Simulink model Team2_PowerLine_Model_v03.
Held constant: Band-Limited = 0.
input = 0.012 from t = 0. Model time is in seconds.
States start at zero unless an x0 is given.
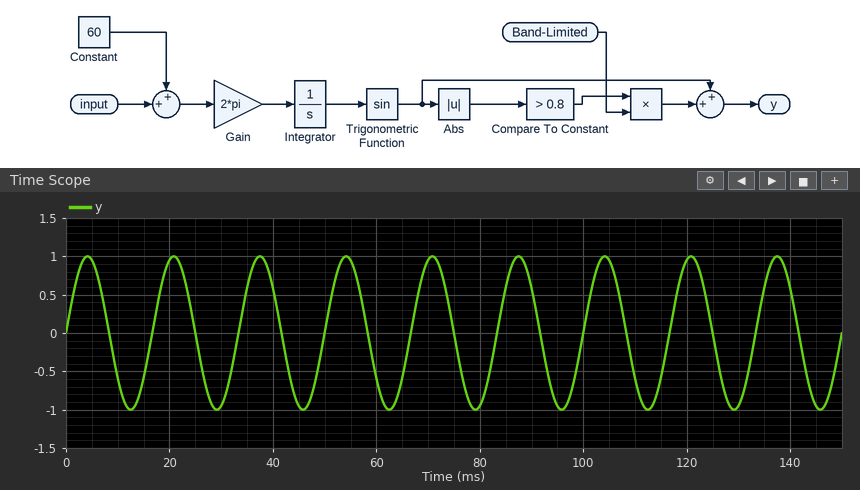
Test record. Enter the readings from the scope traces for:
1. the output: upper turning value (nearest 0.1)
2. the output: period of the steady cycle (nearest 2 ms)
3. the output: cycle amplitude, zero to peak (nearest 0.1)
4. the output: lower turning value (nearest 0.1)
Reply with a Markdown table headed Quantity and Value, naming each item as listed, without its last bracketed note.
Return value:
| Quantity | Value |
|---|---|
| the output: upper turning value | 1.0 |
| the output: period of the steady cycle | 16 ms |
| the output: cycle amplitude, zero to peak | 1.0 |
| the output: lower turning value | -1.0 |
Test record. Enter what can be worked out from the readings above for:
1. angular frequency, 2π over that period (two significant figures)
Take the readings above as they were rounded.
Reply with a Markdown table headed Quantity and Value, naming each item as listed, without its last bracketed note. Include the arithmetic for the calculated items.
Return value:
| Quantity | Value |
|---|---|
| angular frequency, 2π over that period | 2π / 16 = 0.39 rad/ms |
